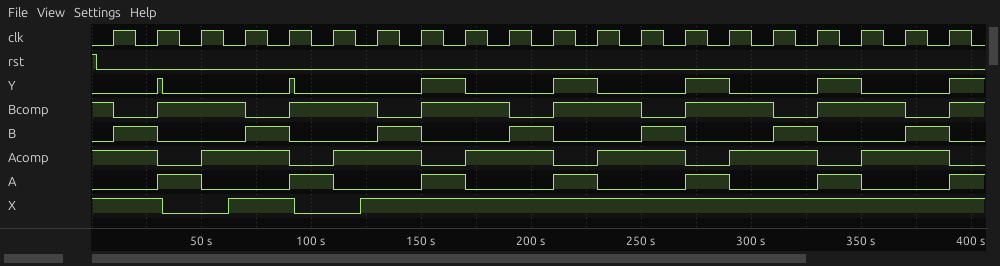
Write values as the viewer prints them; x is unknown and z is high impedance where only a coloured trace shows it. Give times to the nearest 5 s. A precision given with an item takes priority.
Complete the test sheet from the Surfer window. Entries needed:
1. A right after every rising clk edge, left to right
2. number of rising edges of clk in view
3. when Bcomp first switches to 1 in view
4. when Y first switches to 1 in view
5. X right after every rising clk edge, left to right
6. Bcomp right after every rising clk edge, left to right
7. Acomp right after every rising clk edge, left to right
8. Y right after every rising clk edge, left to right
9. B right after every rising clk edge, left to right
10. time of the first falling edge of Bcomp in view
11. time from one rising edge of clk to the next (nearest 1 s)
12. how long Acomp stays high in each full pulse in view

0 1 0 0 1 0 0 1 0 0 1 0 0 1 0 0 1 0 0 1
20
30 s
30 s
1 1 0 1 1 0 1 1 1 1 1 1 1 1 1 1 1 1 1 1
0 1 1 0 1 1 0 1 1 0 1 1 0 1 1 0 1 1 0 1
1 0 1 1 0 1 1 0 1 1 0 1 1 0 1 1 0 1 1 0
0 1 0 0 1 0 0 1 0 0 1 0 0 1 0 0 1 0 0 1
1 0 0 1 0 0 1 0 0 1 0 0 1 0 0 1 0 0 1 0
10 s
20 s
40 s, 40 s, 40 s, 40 s, 40 s, 40 s
